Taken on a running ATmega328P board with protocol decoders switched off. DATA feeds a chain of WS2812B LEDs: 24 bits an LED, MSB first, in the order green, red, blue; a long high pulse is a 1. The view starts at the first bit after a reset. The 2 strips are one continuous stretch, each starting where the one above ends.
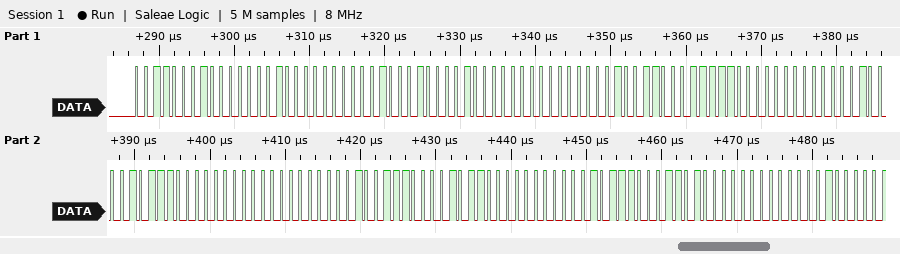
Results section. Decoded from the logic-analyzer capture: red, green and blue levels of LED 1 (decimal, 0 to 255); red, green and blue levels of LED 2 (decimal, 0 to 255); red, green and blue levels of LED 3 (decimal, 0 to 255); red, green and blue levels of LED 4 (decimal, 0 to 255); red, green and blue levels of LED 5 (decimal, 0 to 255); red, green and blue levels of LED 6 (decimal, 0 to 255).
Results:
1, 49, 0
16, 34, 0
31, 19, 0
46, 4, 0
39, 0, 11
23, 0, 26
